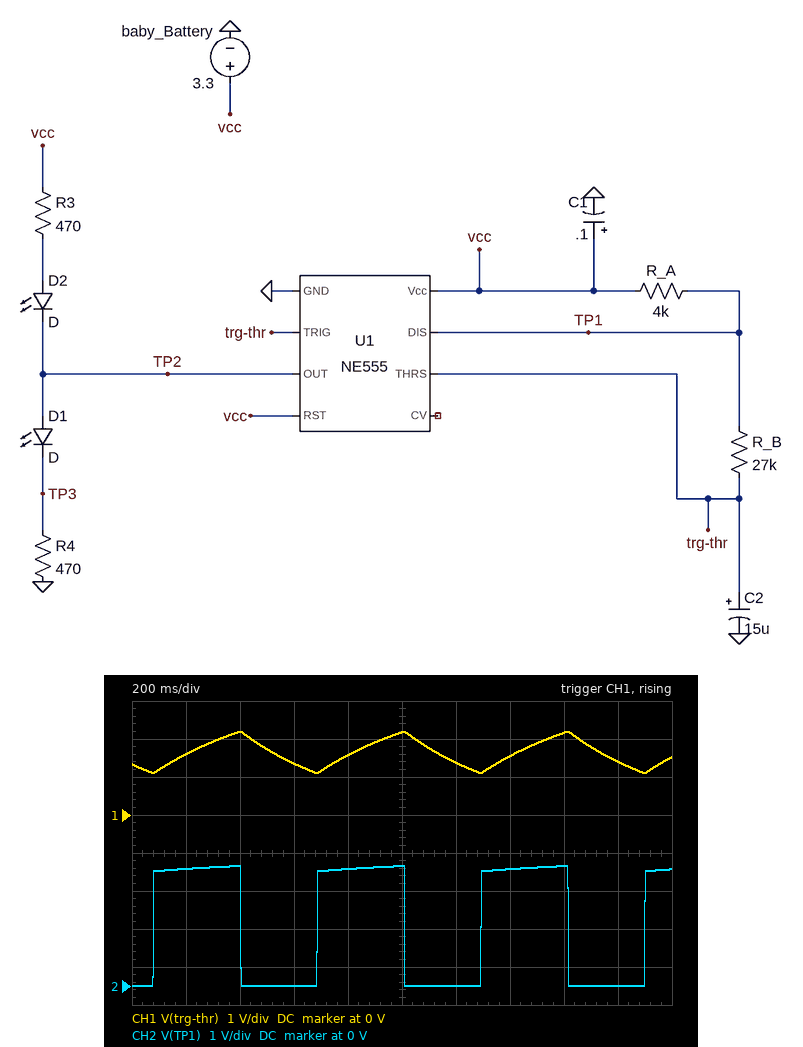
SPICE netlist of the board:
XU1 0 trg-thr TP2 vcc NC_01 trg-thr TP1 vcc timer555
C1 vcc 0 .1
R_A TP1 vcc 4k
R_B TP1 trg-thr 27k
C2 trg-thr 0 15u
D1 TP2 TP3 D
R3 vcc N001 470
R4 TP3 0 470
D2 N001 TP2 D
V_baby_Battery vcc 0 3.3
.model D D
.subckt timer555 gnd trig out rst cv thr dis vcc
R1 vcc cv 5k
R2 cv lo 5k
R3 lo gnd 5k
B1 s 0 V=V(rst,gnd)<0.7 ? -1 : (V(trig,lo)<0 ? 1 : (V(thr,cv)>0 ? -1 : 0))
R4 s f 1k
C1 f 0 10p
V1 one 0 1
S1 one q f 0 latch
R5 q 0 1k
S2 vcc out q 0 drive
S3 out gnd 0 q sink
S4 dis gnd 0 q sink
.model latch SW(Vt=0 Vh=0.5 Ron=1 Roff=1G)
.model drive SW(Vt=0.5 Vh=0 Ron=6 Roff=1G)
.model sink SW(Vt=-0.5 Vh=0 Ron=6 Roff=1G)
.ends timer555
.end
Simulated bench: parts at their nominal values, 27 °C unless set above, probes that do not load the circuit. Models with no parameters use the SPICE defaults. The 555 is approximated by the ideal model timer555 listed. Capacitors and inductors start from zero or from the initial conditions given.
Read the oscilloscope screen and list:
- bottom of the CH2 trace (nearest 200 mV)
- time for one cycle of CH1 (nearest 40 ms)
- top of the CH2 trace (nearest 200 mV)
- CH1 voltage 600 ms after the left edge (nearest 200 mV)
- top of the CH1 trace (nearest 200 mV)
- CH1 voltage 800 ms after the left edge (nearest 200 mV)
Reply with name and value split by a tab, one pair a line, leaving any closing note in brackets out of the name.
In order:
bottom of the CH2 trace	0 V
time for one cycle of CH1	600 ms
top of the CH2 trace	3.2 V
CH1 voltage 600 ms after the left edge	1.4 V
top of the CH1 trace	2.2 V
CH1 voltage 800 ms after the left edge	1.6 V
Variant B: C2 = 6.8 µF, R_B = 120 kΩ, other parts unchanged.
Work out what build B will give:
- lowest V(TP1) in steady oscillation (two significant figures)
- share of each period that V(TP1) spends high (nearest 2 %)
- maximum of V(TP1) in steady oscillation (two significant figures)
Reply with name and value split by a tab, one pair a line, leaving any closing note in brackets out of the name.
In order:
lowest V(TP1) in steady oscillation	5.0 mV
share of each period that V(TP1) spends high	50 %
maximum of V(TP1) in steady oscillation	3.3 V
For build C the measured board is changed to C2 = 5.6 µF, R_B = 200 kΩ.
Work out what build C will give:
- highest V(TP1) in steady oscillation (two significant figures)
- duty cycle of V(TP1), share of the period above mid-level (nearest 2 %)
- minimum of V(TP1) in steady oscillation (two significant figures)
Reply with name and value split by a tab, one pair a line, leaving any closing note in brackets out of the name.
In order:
highest V(TP1) in steady oscillation	3.3 V
duty cycle of V(TP1), share of the period above mid-level	50 %
minimum of V(TP1) in steady oscillation	5.0 mV
